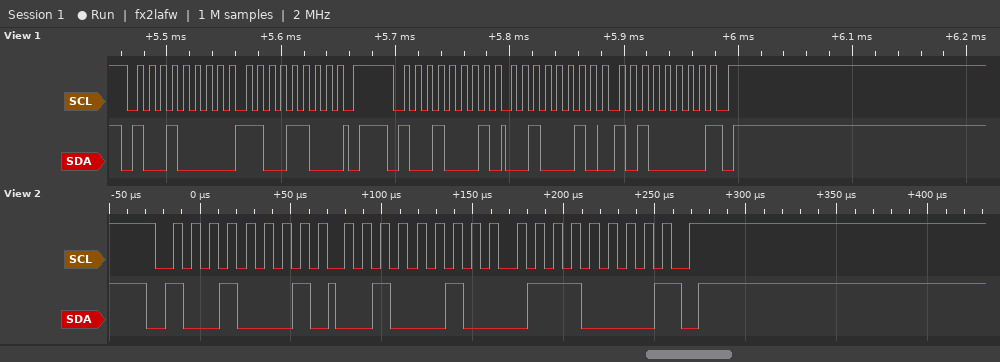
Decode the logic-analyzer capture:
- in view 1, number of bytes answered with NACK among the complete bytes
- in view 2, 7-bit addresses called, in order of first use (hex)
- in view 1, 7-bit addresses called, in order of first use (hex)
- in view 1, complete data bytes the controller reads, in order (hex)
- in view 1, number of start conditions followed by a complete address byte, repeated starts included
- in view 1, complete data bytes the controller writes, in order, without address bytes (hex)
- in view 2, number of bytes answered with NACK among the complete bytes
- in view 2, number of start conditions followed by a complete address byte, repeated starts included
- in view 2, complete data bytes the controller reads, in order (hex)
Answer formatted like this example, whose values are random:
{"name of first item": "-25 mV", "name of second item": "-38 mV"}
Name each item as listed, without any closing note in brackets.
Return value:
{"in view 1, number of bytes answered with NACK among the complete bytes": "1", "in view 2, 7-bit addresses called, in order of first use": "0x48", "in view 1, 7-bit addresses called, in order of first use": "0x48", "in view 1, complete data bytes the controller reads, in order": "22 A0", "in view 1, number of start conditions followed by a complete address byte, repeated starts included": "2", "in view 1, complete data bytes the controller writes, in order, without address bytes": "CC", "in view 2, number of bytes answered with NACK among the complete bytes": "1", "in view 2, number of start conditions followed by a complete address byte, repeated starts included": "1", "in view 2, complete data bytes the controller reads, in order": "22 70"}
